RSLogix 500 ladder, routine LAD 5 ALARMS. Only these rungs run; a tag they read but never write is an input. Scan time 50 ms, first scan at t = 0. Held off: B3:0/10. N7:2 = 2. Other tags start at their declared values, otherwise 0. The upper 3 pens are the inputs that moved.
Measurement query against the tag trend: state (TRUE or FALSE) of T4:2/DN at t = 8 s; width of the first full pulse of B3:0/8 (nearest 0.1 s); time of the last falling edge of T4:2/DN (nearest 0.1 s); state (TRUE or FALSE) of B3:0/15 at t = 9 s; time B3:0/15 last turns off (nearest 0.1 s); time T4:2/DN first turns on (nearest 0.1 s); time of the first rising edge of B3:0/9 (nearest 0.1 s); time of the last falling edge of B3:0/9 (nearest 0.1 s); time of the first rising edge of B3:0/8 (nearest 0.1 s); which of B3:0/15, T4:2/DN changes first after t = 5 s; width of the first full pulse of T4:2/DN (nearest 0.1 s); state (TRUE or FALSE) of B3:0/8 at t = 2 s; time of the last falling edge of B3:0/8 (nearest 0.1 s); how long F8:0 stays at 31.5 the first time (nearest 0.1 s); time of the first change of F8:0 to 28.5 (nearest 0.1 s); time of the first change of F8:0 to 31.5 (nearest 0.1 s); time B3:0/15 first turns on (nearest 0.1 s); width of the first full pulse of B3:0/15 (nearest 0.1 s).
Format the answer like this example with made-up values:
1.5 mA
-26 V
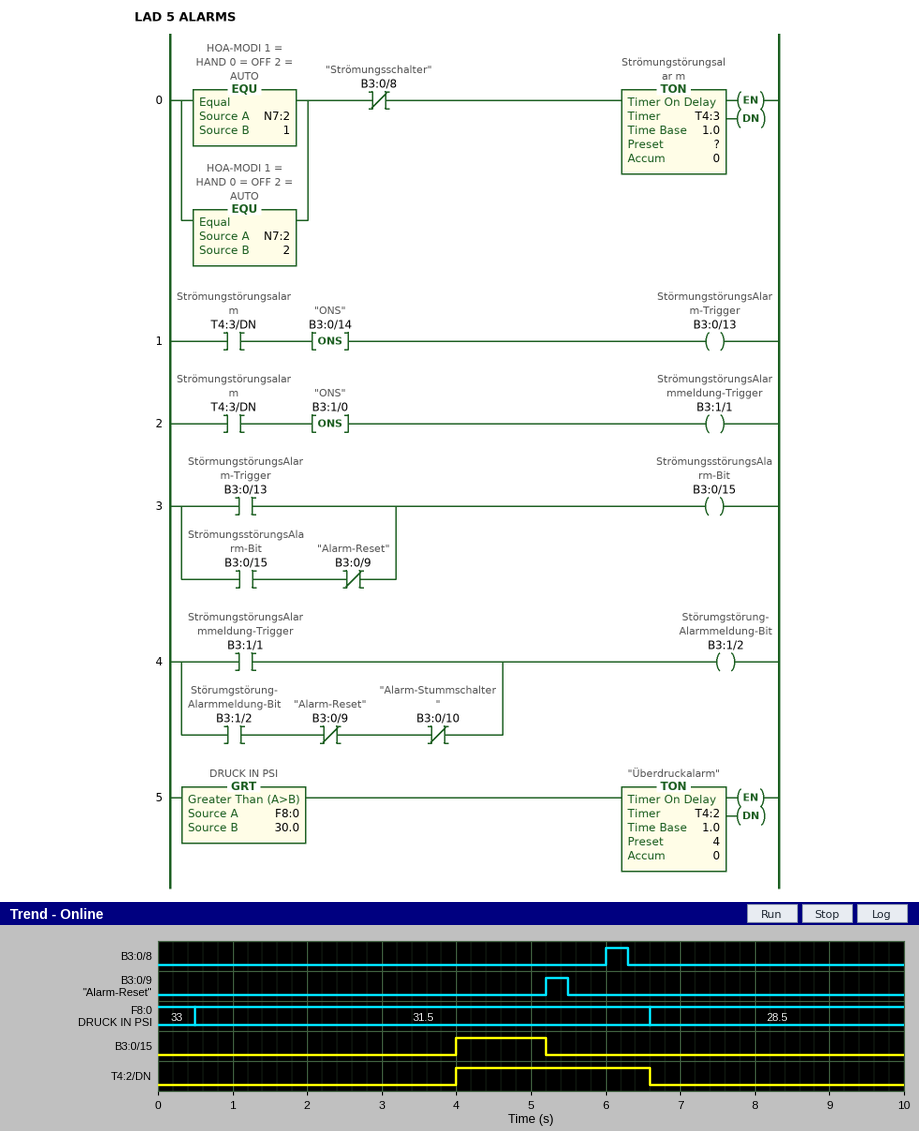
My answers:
FALSE
0.3 s
6.6 s
FALSE
5.2 s
4.0 s
5.2 s
5.5 s
6.0 s
B3:0/15
2.6 s
FALSE
6.3 s
6.1 s
6.6 s
0.5 s
4.0 s
1.2 s
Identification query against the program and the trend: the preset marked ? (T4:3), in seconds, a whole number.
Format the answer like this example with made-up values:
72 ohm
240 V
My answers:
4 s
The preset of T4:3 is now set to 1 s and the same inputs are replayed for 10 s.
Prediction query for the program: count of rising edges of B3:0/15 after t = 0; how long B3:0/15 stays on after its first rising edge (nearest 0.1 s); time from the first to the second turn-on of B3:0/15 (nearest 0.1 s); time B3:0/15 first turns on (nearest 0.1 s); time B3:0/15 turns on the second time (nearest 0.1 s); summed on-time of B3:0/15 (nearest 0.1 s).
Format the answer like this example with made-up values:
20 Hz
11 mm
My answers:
2
4.2 s
6.3 s
1.0 s
7.3 s
6.9 s
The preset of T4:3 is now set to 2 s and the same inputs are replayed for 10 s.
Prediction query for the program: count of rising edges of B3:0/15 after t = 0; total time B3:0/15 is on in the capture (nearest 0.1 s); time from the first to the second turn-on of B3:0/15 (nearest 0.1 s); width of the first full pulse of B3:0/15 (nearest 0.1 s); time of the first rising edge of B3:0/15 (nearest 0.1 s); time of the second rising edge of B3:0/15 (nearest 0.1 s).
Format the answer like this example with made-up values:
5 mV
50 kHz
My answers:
2
4.9 s
6.3 s
3.2 s
2.0 s
8.3 s
